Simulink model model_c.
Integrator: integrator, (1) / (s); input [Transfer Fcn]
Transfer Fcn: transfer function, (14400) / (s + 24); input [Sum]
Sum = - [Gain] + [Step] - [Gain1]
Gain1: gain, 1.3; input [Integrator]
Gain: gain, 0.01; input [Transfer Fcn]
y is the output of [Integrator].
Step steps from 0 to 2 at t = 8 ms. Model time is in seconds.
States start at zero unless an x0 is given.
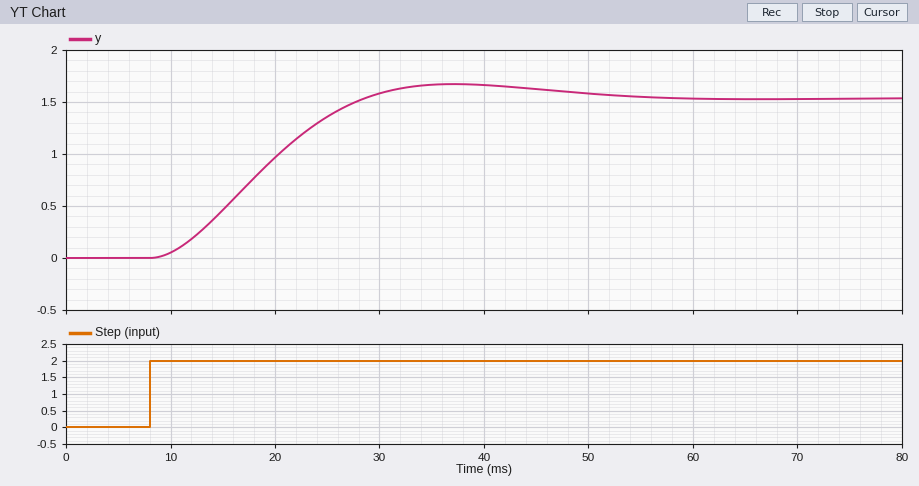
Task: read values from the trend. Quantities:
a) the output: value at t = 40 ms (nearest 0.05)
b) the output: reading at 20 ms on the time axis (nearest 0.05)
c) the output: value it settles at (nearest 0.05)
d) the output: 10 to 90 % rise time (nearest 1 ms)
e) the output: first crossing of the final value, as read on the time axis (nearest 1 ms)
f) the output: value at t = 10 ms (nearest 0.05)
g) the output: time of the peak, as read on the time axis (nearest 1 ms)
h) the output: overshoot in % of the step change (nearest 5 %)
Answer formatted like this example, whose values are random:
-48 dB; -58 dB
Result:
1.65; 0.95; 1.55; 14 ms; 29 ms; 0.05; 37 ms; 10 %
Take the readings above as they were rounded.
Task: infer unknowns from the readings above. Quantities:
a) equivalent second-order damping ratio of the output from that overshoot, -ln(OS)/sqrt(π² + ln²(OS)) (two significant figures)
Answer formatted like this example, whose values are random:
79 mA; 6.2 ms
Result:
0.59
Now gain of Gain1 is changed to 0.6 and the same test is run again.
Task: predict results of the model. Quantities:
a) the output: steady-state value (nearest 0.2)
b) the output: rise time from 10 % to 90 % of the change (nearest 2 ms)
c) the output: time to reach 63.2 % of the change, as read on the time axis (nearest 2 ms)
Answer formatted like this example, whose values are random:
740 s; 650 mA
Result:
3.4; 32 ms; 30 ms
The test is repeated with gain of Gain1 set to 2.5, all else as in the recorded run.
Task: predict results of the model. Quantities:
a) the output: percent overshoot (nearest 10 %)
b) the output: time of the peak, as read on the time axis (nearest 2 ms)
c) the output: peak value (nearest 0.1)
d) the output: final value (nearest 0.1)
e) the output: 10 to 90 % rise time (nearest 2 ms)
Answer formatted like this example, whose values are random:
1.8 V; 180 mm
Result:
20 %; 26 ms; 1.0; 0.8; 8 ms
